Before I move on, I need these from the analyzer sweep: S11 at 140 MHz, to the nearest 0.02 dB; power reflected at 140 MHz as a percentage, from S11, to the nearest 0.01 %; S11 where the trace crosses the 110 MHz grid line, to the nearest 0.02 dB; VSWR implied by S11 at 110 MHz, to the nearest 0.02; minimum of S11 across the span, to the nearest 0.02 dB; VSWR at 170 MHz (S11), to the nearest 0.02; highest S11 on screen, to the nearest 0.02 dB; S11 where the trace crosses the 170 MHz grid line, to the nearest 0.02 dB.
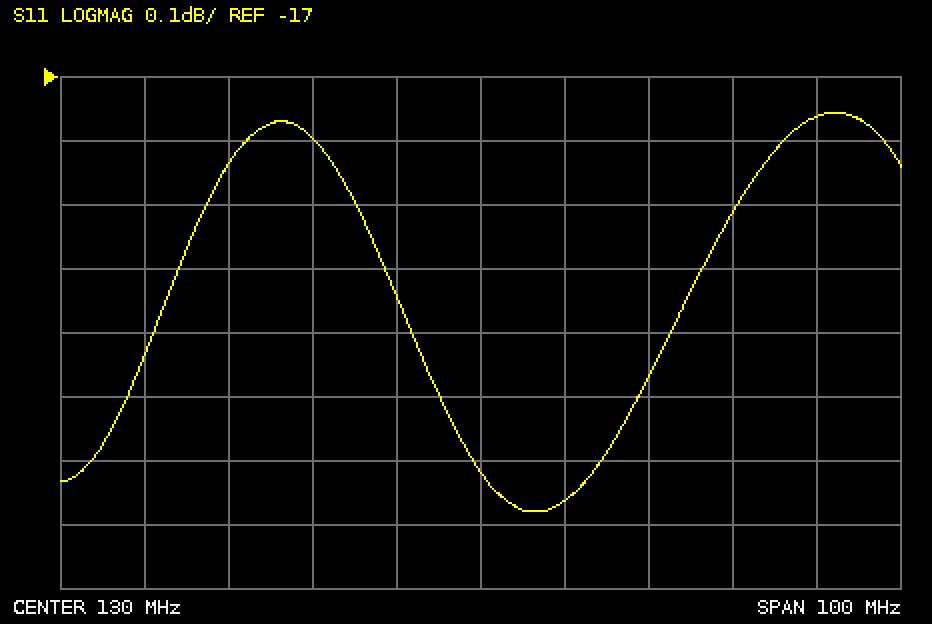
-17.66 dB
1.71 %
-17.10 dB
1.32
-17.68 dB
1.32
-17.06 dB
-17.06 dB
